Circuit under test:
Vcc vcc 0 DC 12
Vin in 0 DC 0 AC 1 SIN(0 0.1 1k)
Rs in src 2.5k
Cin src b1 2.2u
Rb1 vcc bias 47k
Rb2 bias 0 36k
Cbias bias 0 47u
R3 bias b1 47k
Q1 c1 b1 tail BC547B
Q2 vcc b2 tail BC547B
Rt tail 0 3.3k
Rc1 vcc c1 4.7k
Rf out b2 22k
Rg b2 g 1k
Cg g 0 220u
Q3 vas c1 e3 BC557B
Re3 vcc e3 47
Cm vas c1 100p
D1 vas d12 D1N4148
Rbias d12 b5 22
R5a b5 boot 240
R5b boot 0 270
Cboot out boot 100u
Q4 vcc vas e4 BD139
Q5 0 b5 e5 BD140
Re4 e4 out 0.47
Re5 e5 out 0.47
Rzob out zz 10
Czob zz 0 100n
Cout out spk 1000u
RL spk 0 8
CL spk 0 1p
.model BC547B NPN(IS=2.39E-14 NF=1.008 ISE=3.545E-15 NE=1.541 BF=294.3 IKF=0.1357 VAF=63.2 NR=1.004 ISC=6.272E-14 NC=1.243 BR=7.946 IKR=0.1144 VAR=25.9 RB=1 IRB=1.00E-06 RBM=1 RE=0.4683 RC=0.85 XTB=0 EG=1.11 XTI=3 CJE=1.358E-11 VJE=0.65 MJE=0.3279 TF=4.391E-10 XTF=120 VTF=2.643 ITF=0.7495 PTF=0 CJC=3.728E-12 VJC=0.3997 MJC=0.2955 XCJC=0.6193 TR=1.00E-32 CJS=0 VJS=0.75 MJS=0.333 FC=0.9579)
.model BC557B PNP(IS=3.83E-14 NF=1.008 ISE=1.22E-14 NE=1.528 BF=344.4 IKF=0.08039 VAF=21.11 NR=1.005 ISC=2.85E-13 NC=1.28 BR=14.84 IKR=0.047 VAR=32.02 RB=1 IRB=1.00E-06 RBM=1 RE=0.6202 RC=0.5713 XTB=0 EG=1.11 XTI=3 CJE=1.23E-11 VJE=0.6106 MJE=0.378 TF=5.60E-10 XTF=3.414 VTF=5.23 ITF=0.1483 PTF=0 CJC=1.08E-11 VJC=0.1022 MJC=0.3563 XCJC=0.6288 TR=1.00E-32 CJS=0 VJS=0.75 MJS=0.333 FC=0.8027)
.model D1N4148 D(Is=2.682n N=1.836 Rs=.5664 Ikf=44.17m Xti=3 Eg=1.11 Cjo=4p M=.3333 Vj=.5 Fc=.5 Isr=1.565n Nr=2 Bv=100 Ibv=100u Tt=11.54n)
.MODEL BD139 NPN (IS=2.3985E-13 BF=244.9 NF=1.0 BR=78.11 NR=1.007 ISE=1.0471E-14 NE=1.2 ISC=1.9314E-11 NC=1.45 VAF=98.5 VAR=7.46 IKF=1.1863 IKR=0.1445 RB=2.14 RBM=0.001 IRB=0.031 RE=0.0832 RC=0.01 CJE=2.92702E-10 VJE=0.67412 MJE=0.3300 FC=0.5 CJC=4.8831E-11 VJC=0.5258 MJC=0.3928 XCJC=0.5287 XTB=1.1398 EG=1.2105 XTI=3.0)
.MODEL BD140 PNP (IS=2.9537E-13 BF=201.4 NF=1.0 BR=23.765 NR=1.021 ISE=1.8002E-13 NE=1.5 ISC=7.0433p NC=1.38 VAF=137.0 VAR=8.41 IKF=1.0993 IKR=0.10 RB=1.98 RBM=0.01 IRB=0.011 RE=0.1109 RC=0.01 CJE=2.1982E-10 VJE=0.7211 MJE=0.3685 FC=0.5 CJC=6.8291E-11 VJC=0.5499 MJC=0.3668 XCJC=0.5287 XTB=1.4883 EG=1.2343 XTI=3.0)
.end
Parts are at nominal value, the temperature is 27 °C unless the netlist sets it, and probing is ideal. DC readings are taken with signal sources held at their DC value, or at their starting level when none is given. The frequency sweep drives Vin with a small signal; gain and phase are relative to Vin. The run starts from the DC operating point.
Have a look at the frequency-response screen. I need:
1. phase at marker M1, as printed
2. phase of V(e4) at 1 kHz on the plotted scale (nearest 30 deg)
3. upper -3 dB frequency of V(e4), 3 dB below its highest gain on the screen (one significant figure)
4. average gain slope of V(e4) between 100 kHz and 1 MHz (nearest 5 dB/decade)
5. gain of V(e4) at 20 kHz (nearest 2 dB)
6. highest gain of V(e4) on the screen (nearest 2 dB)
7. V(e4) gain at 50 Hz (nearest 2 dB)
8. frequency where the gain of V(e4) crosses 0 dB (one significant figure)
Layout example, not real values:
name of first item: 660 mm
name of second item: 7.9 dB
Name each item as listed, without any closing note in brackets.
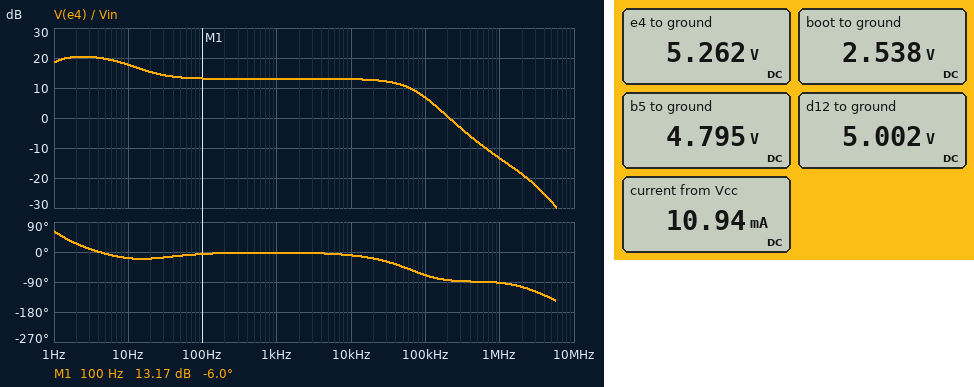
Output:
phase at marker M1, as printed: -6.0 deg
phase of V(e4) at 1 kHz on the plotted scale: 0 deg
upper -3 dB frequency of V(e4), 3 dB below its highest gain on the screen: 10 Hz
average gain slope of V(e4) between 100 kHz and 1 MHz: -20 dB/decade
gain of V(e4) at 20 kHz: 12 dB
highest gain of V(e4) on the screen: 20 dB
V(e4) gain at 50 Hz: 14 dB
frequency where the gain of V(e4) crosses 0 dB: 200 kHz
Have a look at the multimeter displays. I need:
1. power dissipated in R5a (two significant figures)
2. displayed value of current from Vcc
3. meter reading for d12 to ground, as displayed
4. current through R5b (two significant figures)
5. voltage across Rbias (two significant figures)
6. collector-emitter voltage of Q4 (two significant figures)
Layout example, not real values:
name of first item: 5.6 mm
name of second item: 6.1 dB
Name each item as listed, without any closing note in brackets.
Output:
power dissipated in R5a: 21 mW
displayed value of current from Vcc: 10.94 mA
meter reading for d12 to ground, as displayed: 5.002 V
current through R5b: 9.4 mA
voltage across Rbias: 210 mV
collector-emitter voltage of Q4: 6.7 V
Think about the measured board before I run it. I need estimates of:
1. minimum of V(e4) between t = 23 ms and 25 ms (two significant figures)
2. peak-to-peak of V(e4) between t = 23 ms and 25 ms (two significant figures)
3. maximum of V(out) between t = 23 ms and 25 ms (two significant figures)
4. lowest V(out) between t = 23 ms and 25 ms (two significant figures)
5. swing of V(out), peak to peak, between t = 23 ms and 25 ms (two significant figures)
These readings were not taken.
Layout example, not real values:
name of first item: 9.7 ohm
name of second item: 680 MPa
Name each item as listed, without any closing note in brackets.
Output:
minimum of V(e4) between t = 23 ms and 25 ms: 3.2 V
peak-to-peak of V(e4) between t = 23 ms and 25 ms: 4.2 V
maximum of V(out) between t = 23 ms and 25 ms: 7.3 V
lowest V(out) between t = 23 ms and 25 ms: 3.2 V
swing of V(out), peak to peak, between t = 23 ms and 25 ms: 4.1 V
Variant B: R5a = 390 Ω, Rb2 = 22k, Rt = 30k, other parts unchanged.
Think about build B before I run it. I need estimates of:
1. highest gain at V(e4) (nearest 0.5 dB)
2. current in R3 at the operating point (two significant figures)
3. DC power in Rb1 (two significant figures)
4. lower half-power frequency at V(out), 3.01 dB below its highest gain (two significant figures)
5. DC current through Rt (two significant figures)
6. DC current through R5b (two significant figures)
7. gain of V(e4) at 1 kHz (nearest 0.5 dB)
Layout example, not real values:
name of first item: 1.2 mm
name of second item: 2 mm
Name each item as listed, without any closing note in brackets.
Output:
highest gain at V(e4): -56.5 dB
current in R3 at the operating point: 340 nA
DC power in Rb1: 1.4 mW
lower half-power frequency at V(out), 3.01 dB below its highest gain: 1.1 Hz
DC current through Rt: 110 µA
DC current through R5b: 14 µA
gain of V(e4) at 1 kHz: -64.5 dB
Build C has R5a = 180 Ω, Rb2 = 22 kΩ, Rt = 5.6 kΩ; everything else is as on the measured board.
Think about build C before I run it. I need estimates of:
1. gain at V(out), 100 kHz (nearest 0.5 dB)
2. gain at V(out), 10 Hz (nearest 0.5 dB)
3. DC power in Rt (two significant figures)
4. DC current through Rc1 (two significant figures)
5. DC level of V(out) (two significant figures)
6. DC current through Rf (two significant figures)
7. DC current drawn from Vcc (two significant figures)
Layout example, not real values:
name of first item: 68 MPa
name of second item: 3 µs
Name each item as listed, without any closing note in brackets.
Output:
gain at V(out), 100 kHz: 2.5 dB
gain at V(out), 10 Hz: 13.0 dB
DC power in Rt: 1.8 mW
DC current through Rc1: 220 µA
DC level of V(out): 3.8 V
DC current through Rf: 1.0 µA
DC current drawn from Vcc: 8.2 mA
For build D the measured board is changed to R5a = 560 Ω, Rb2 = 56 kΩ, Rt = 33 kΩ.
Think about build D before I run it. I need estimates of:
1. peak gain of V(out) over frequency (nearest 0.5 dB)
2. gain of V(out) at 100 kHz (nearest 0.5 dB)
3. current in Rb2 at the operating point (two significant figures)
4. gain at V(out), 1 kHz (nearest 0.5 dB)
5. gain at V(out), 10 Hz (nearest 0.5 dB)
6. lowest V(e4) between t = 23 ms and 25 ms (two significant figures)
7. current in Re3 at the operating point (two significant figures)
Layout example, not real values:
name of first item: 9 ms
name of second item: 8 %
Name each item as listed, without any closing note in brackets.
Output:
peak gain of V(out) over frequency: -28.0 dB
gain of V(out) at 100 kHz: -48.5 dB
current in Rb2 at the operating point: 120 µA
gain at V(out), 1 kHz: -36.0 dB
gain at V(out), 10 Hz: -31.0 dB
lowest V(e4) between t = 23 ms and 25 ms: 3.0 V
current in Re3 at the operating point: 3.2 mA
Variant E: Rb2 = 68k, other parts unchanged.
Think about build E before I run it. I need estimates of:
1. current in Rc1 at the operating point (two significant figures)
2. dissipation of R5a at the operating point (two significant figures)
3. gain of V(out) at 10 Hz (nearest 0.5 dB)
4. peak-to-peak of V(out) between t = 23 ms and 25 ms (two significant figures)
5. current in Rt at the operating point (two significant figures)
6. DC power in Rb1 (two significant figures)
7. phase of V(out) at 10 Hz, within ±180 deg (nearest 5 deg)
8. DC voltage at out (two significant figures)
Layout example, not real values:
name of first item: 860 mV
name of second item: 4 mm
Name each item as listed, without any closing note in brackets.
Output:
current in Rc1 at the operating point: 280 µA
dissipation of R5a at the operating point: 41 mW
gain of V(out) at 10 Hz: 24.5 dB
peak-to-peak of V(out) between t = 23 ms and 25 ms: 4.1 V
current in Rt at the operating point: 1.9 mA
DC power in Rb1: 520 µW
phase of V(out) at 10 Hz, within ±180 deg: -5 deg
DC voltage at out: 7.2 V
